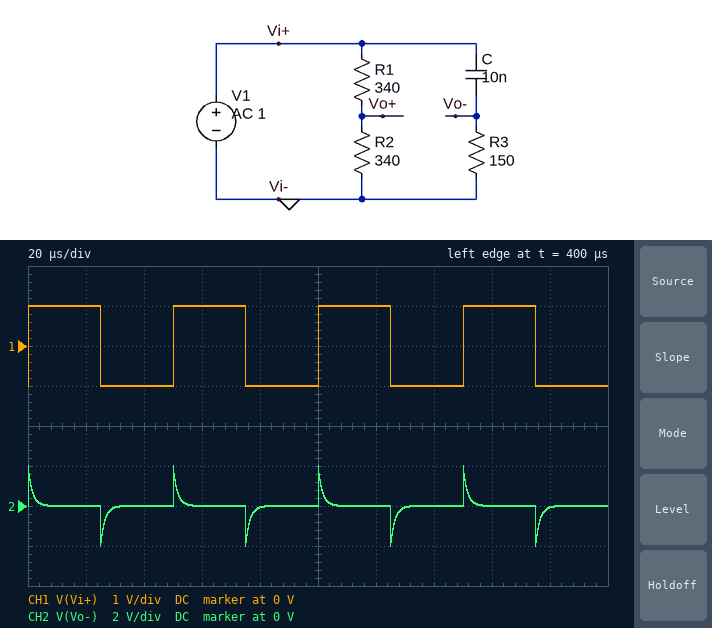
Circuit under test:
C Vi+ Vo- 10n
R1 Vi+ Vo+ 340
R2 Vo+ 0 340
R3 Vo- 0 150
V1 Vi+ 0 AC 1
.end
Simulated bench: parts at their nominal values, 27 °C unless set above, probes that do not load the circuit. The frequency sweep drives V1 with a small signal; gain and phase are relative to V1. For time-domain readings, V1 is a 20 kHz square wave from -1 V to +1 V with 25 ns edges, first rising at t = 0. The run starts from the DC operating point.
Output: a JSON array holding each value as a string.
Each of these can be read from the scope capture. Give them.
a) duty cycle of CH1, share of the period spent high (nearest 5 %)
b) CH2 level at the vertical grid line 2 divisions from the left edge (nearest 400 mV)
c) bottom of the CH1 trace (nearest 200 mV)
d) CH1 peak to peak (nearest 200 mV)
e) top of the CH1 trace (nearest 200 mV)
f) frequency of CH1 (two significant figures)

["50 %", "0 V", "-1.0 V", "2.0 V", "1.0 V", "20 kHz"]
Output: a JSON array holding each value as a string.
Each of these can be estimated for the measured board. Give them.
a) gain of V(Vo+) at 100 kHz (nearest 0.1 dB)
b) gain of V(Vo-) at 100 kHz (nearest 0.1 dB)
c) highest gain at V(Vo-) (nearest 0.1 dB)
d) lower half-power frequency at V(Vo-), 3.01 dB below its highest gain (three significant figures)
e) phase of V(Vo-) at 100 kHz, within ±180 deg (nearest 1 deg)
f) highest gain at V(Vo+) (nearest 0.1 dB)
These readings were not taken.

["-6.0 dB", "-3.3 dB", "0 dB", "106 kHz", "47 deg", "-6.0 dB"]
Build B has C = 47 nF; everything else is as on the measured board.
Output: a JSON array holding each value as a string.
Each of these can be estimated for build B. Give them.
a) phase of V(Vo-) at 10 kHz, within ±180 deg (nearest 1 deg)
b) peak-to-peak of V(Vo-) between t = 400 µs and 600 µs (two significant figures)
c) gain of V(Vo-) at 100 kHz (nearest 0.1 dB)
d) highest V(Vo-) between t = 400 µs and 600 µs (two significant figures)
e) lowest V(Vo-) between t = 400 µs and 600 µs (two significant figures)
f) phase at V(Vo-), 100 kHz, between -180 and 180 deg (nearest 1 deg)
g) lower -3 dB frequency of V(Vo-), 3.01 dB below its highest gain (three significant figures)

["66 deg", "3.9 V", "-0.2 dB", "1.9 V", "-1.9 V", "13 deg", "22.6 kHz"]
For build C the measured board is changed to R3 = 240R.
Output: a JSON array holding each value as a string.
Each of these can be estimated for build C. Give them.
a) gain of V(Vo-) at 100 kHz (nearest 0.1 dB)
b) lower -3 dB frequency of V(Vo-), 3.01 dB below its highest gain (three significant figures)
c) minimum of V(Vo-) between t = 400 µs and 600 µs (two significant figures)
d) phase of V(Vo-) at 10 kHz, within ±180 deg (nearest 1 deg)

["-1.6 dB", "66.3 kHz", "-2.0 V", "81 deg"]
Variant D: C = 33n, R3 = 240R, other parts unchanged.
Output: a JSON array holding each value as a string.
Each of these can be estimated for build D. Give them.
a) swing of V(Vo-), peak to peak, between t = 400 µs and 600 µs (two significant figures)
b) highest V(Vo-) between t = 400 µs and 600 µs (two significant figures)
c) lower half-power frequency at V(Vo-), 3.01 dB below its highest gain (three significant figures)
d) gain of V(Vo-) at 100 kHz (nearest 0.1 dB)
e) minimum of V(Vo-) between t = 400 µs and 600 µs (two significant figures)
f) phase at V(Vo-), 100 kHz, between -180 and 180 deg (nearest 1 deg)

["3.8 V", "1.9 V", "20.1 kHz", "-0.2 dB", "-1.9 V", "11 deg"]
